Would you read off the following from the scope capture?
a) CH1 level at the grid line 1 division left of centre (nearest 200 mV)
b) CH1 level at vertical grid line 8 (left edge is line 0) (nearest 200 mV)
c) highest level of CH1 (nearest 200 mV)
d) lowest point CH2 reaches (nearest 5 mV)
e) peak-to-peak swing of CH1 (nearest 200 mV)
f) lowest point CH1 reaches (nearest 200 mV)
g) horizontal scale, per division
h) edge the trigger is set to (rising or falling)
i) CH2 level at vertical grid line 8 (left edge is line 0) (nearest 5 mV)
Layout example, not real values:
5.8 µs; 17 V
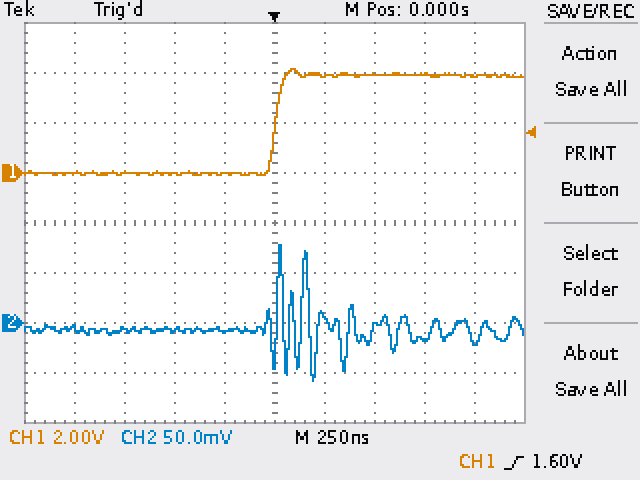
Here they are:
0.0 V; 4.0 V; 4.2 V; -60 mV; 4.2 V; 0.0 V; 250 ns; rising; -15 mV
